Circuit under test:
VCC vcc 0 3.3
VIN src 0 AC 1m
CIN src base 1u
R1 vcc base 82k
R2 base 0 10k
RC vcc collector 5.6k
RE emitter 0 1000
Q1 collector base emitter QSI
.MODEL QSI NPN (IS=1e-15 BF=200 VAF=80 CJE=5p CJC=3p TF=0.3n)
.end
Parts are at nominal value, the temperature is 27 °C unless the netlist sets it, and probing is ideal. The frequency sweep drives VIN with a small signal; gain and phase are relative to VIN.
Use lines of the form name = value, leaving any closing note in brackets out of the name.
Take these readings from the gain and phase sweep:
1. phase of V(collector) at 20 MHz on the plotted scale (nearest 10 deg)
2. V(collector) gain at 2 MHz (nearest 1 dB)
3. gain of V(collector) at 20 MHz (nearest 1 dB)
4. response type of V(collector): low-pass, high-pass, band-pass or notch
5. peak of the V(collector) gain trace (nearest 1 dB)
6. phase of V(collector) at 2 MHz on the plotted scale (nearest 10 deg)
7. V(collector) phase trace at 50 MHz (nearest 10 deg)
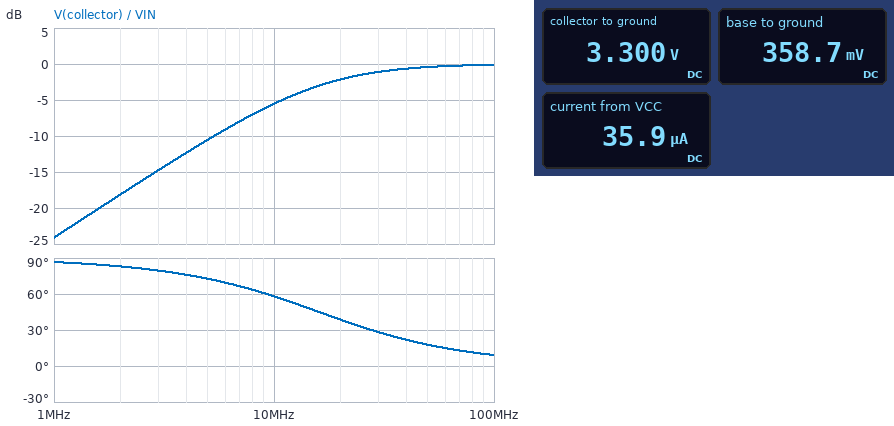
phase of V(collector) at 20 MHz on the plotted scale = 40 deg
V(collector) gain at 2 MHz = -18 dB
gain of V(collector) at 20 MHz = -2 dB
response type of V(collector): low-pass, high-pass, band-pass or notch = high-pass
peak of the V(collector) gain trace = 0 dB
phase of V(collector) at 2 MHz on the plotted scale = 80 deg
V(collector) phase trace at 50 MHz = 20 deg
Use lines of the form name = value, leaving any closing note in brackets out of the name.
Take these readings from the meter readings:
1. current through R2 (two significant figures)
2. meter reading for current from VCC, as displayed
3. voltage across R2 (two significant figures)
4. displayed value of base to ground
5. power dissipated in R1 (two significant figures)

current through R2 = 36 µA
meter reading for current from VCC, as displayed = 35.9 µA
voltage across R2 = 360 mV
displayed value of base to ground = 358.7 mV
power dissipated in R1 = 110 µW
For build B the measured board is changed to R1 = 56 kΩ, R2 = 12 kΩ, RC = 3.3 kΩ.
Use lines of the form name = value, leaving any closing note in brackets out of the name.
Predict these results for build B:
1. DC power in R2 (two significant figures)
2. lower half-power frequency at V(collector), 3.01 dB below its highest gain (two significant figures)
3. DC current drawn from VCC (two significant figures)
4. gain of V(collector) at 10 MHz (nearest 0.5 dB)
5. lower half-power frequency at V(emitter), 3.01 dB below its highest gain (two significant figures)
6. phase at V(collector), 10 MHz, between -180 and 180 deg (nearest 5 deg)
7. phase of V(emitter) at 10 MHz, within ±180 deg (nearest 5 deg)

DC power in R2 = 28 µW
lower half-power frequency at V(collector), 3.01 dB below its highest gain = 11 MHz
DC current drawn from VCC = 54 µA
gain of V(collector) at 10 MHz = -3.5 dB
lower half-power frequency at V(emitter), 3.01 dB below its highest gain = 25 MHz
phase at V(collector), 10 MHz, between -180 and 180 deg = 110 deg
phase of V(emitter) at 10 MHz, within ±180 deg = 45 deg
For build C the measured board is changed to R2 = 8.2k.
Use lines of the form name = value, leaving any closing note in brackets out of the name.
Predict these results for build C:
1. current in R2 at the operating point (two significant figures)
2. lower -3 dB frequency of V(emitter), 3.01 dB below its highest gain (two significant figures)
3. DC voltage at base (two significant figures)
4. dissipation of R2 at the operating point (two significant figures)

current in R2 at the operating point = 37 µA
lower -3 dB frequency of V(emitter), 3.01 dB below its highest gain = 27 MHz
DC voltage at base = 300 mV
dissipation of R2 at the operating point = 11 µW
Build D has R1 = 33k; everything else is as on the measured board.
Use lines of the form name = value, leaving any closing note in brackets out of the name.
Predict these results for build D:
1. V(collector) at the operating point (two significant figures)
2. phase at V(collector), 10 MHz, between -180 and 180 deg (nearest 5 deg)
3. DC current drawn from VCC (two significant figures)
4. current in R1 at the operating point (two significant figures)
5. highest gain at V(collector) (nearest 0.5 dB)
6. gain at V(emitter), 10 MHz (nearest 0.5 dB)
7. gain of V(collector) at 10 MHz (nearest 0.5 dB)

V(collector) at the operating point = 2.7 V
phase at V(collector), 10 MHz, between -180 and 180 deg = 130 deg
DC current drawn from VCC = 180 µA
current in R1 at the operating point = 77 µA
highest gain at V(collector) = 13.0 dB
gain at V(emitter), 10 MHz = -2.0 dB
gain of V(collector) at 10 MHz = 11.5 dB
